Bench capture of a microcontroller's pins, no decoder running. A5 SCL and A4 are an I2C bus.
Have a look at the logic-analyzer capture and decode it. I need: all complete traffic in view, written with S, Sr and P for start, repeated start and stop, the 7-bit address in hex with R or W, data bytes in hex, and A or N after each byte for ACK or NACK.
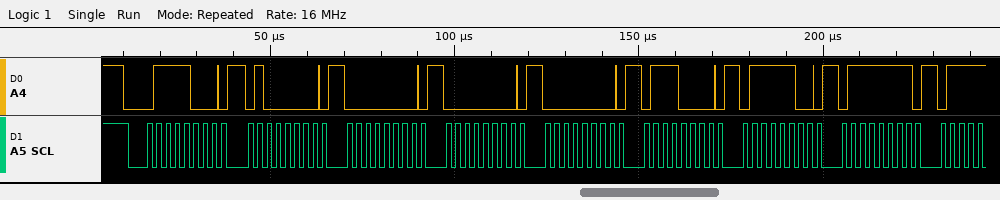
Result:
S 3CW A 40 A 00 A 00 A 00 A 70 A 7C A 7F A
